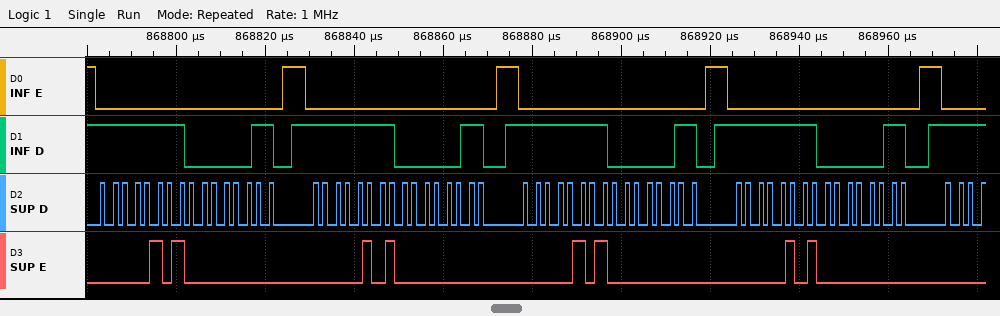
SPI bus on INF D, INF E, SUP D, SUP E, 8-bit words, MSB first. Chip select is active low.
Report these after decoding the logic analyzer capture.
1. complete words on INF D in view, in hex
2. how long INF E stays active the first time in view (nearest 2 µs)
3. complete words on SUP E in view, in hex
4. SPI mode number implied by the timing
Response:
FF, 03, FF, 03, FF, 03, FF, 03
42 µs
05, 00, 05, 00, 05, 00, 05, 00
0
